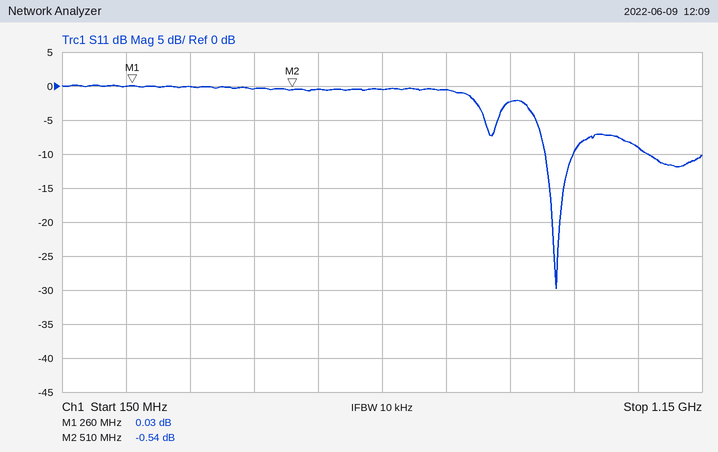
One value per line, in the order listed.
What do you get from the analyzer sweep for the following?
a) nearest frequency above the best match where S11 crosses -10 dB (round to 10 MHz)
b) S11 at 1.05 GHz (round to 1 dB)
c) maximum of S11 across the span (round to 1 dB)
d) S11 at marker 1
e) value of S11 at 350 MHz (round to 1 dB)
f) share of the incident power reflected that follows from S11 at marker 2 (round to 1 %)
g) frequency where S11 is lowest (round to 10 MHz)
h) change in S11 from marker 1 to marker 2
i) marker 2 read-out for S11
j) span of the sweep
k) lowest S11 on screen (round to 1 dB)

950 MHz
-9 dB
0 dB
0.03 dB
0 dB
88 %
920 MHz
-0.57 dB
-0.54 dB
1 GHz
-30 dB
